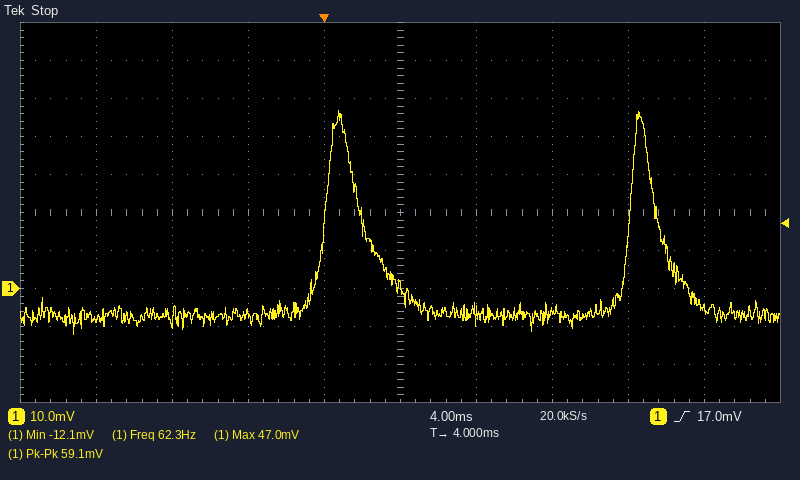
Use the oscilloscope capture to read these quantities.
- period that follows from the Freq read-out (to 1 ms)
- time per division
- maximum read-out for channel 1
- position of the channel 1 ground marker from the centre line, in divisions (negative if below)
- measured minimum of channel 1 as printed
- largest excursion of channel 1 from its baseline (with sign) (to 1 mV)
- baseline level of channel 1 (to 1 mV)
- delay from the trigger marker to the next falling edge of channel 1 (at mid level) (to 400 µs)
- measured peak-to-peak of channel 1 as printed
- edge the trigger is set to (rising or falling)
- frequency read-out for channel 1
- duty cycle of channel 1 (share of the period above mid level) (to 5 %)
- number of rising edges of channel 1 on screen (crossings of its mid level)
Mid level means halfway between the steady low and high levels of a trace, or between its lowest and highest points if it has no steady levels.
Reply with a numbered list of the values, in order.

1. 16 ms
2. 4 ms
3. 47.0 mV
4. -2.0 div
5. -12.1 mV
6. +54 mV
7. -7 mV
8. 2.0 ms
9. 59.1 mV
10. rising
11. 62.3 Hz
12. 10 %
13. 2
